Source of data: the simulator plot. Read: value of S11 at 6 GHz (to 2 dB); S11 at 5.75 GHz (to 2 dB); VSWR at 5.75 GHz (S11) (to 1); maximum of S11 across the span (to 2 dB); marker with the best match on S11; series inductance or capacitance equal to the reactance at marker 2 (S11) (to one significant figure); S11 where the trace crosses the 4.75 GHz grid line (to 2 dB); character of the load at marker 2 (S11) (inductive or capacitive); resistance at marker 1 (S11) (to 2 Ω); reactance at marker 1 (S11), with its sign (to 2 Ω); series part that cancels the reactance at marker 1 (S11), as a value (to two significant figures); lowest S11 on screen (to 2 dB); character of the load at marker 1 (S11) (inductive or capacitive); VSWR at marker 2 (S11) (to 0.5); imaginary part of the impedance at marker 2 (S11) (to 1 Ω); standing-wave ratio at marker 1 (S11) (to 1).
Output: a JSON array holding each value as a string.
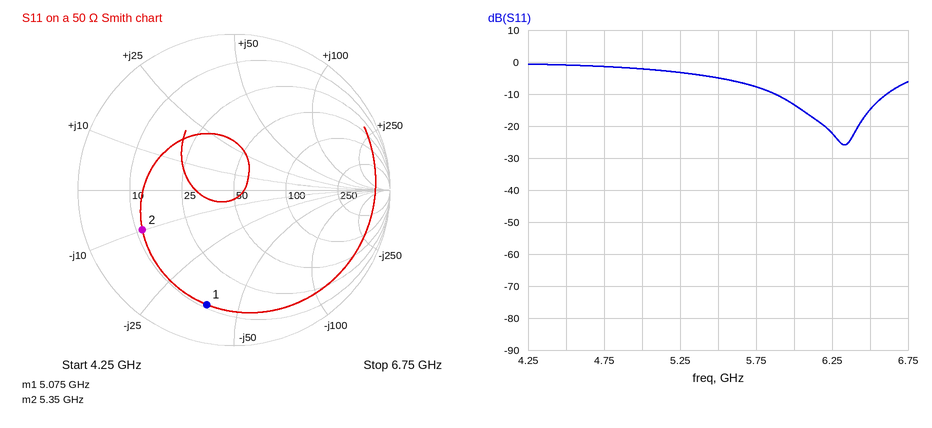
["-14 dB", "-8 dB", "2", "0 dB", "marker 2", "3 pF", "-2 dB", "capacitive", "12 Ω", "-38 Ω", "1.2 nH", "-26 dB", "capacitive", "4.5", "-10 Ω", "7"]
